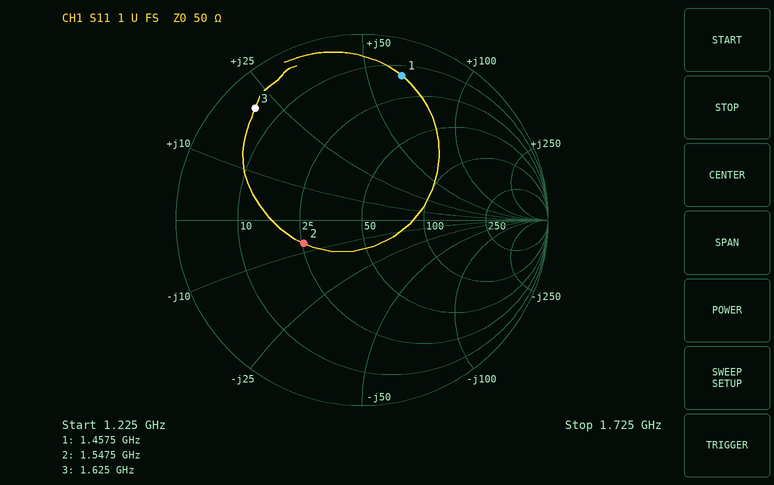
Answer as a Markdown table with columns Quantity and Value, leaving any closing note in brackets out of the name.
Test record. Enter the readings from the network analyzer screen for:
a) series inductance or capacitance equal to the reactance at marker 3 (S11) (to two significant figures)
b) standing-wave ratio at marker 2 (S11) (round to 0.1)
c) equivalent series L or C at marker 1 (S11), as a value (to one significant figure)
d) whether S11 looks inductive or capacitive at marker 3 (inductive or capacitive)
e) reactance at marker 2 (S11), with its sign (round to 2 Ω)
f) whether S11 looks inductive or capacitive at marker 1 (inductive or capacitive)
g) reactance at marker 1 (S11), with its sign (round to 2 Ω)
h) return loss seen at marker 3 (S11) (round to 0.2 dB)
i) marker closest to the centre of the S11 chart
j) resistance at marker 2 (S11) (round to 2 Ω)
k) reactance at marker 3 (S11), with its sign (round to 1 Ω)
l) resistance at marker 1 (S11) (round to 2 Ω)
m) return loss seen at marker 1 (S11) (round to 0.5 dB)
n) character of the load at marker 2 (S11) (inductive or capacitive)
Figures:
| Quantity | Value |
|---|---|
| series inductance or capacitance equal to the reactance at marker 3 (S11) | 2.1 nH |
| standing-wave ratio at marker 2 (S11) | 2.0 |
| equivalent series L or C at marker 1 (S11), as a value | 7 nH |
| whether S11 looks inductive or capacitive at marker 3 | inductive |
| reactance at marker 2 (S11), with its sign | -8 Ω |
| whether S11 looks inductive or capacitive at marker 1 | inductive |
| reactance at marker 1 (S11), with its sign | +64 Ω |
| return loss seen at marker 3 (S11) | 1.6 dB |
| marker closest to the centre of the S11 chart | marker 2 |
| resistance at marker 2 (S11) | 26 Ω |
| reactance at marker 3 (S11), with its sign | +21 Ω |
| resistance at marker 1 (S11) | 14 Ω |
| return loss seen at marker 1 (S11) | 2.0 dB |
| character of the load at marker 2 (S11) | capacitive |
